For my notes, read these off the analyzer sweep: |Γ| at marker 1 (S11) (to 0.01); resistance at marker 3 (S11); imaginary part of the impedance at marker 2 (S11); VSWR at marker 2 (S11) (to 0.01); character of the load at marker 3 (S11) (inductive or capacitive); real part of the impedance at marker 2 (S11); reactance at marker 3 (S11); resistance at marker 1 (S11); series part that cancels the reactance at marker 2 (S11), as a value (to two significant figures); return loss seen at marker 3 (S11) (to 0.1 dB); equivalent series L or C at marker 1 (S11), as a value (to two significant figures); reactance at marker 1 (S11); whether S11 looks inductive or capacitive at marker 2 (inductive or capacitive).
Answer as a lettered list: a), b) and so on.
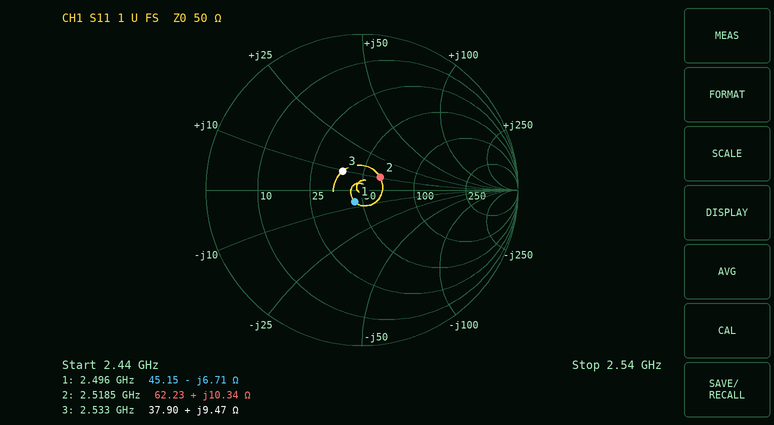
a) 0.09
b) 37.90 Ω
c) +10.34 Ω
d) 1.33
e) inductive
f) 62.23 Ω
g) +9.47 Ω
h) 45.15 Ω
i) 6.1 pF
j) 15.2 dB
k) 9.5 pF
l) -6.71 Ω
m) inductive
